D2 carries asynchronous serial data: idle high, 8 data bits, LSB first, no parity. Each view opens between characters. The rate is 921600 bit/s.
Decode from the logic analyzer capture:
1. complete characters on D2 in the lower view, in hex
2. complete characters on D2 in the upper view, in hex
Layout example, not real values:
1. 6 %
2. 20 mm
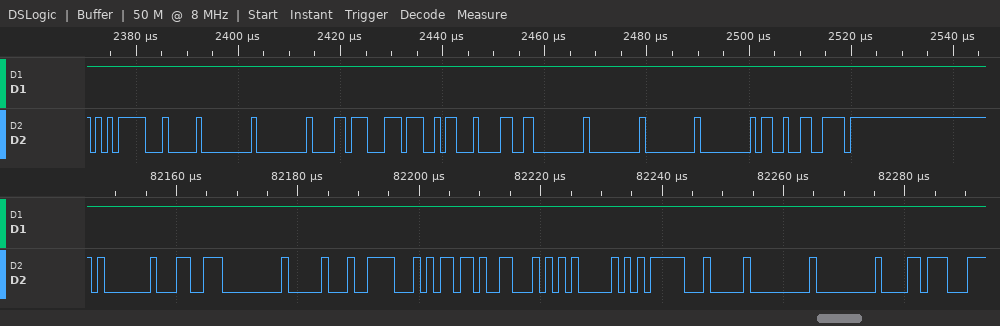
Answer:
1. 01, CC, 00, 10, 1E, 6D, 46, 05, F5, 04, 00, 00, D8
2. F5, 04, 00, 00, D8, DC, 1A, 98, 00, 00, 00, 00, 93, DE
